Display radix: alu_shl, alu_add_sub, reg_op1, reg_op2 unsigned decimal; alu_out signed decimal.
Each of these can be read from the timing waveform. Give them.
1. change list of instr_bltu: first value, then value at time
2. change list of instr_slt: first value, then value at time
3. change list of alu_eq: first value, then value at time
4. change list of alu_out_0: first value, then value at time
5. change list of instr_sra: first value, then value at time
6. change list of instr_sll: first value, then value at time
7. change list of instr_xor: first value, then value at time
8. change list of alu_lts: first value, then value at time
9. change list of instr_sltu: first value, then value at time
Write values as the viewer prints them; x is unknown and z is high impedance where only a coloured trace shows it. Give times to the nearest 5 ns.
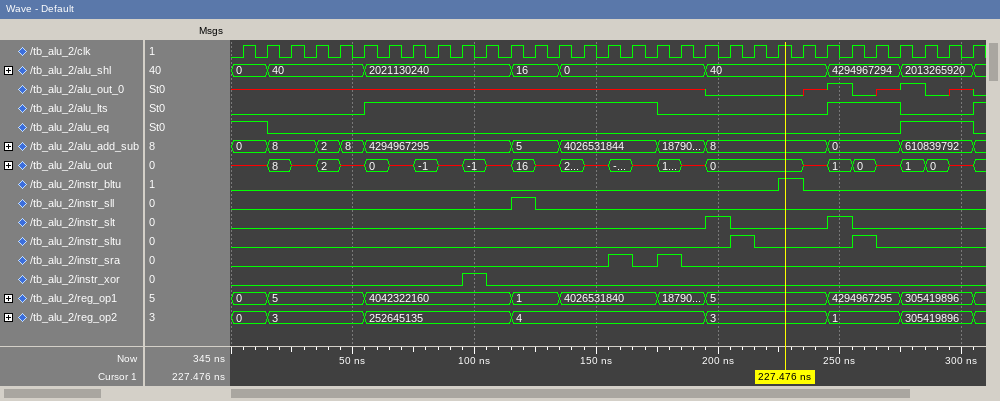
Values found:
0, 1 at 225 ns, 0 at 235 ns
0, 1 at 195 ns, 0 at 205 ns, 1 at 245 ns, 0 at 255 ns
1, 0 at 15 ns, 1 at 275 ns, 0 at 305 ns
x, 0 at 195 ns, x at 235 ns, 1 at 245 ns, 0 at 255 ns, x at 265 ns, 1 at 275 ns, 0 at 285 ns, x at 295 ns, 0 at 305 ns
0, 1 at 155 ns, 0 at 165 ns, 1 at 175 ns, 0 at 185 ns
0, 1 at 115 ns, 0 at 125 ns
0, 1 at 95 ns, 0 at 105 ns
0, 1 at 55 ns, 0 at 175 ns, 1 at 245 ns, 0 at 275 ns, 1 at 305 ns
0, 1 at 205 ns, 0 at 215 ns, 1 at 255 ns, 0 at 265 ns
